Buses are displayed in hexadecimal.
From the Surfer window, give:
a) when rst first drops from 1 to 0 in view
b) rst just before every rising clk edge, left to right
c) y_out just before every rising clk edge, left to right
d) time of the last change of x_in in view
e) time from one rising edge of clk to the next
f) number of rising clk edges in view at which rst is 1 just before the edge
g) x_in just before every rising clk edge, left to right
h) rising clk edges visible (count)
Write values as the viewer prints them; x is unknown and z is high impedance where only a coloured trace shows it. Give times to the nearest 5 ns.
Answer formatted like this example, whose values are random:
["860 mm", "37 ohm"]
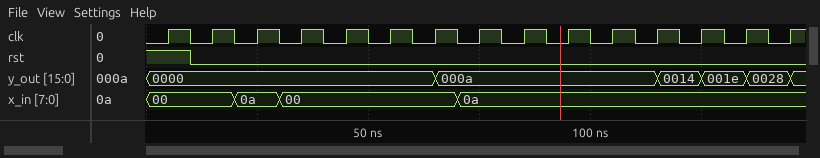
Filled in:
["10 ns", "1 0 0 0 0 0 0 0 0 0 0 0 0 0 0", "0000, 0000, 0000, 0000, 0000, 0000, 0000, 000a, 000a, 000a, 000a, 000a, 0014, 001e, 0028", "70 ns", "10 ns", "1", "00, 00, 0a, 00, 00, 00, 00, 0a, 0a, 0a, 0a, 0a, 0a, 0a, 0a", "15"]
